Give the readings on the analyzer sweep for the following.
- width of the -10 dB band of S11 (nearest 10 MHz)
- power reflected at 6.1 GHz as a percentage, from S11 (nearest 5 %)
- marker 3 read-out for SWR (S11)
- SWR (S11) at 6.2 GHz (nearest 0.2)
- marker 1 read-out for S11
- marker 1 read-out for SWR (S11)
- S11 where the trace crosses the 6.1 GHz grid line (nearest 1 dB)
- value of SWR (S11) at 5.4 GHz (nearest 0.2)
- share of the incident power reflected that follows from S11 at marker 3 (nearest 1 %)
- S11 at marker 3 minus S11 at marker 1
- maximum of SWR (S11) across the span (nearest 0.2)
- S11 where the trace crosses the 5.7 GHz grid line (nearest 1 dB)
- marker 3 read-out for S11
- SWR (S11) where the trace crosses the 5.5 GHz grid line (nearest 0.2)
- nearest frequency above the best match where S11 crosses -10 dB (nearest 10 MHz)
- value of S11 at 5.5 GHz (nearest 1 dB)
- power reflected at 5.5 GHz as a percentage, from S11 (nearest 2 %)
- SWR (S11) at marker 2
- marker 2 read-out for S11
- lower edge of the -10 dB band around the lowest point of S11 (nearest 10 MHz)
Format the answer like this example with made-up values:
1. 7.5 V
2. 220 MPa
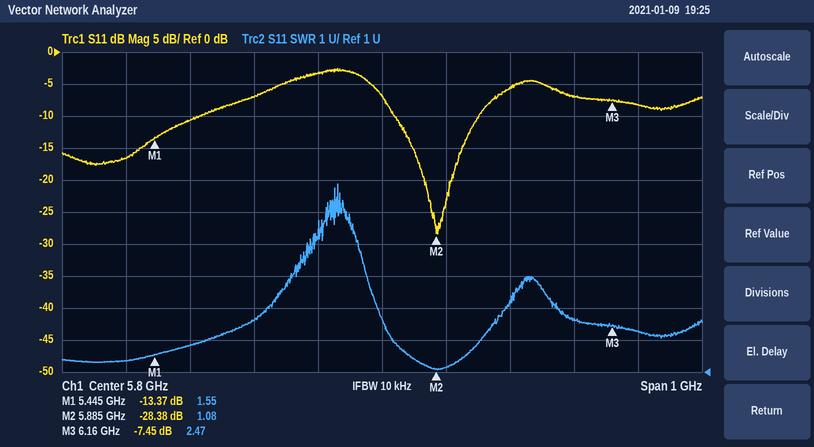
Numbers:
1. 130 MHz
2. 20 %
3. 2.47
4. 2.2
5. -13.37 dB
6. 1.55
7. -7 dB
8. 1.4
9. 18 %
10. 5.92 dB
11. 6.8
12. -3 dB
13. -7.45 dB
14. 1.8
15. 5.95 GHz
16. -11 dB
17. 8 %
18. 1.08
19. -28.38 dB
20. 5.82 GHz
